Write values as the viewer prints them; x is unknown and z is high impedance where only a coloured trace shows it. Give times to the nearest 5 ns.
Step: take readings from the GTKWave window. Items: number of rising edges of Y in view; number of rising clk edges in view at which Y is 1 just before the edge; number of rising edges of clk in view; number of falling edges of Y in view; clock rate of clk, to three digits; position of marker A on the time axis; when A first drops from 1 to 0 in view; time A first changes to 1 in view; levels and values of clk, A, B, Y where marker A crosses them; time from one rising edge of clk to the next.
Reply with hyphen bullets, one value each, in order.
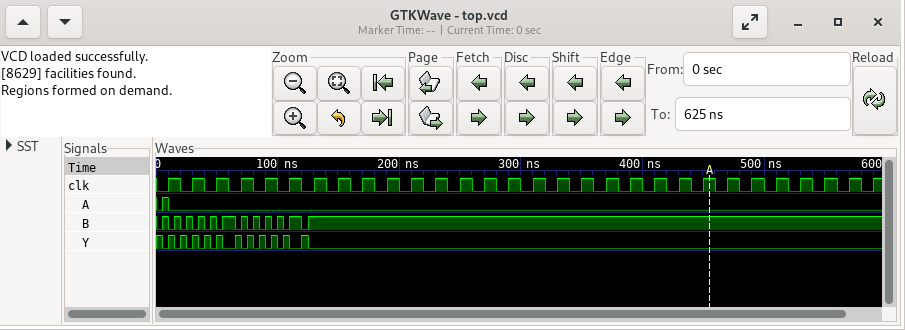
- 11
- 3
- 30
- 12
- 50.0 MHz
- 455 ns
- 10 ns
- 5 ns
- clk=1, A=0, B=1, Y=0
- 20 ns
